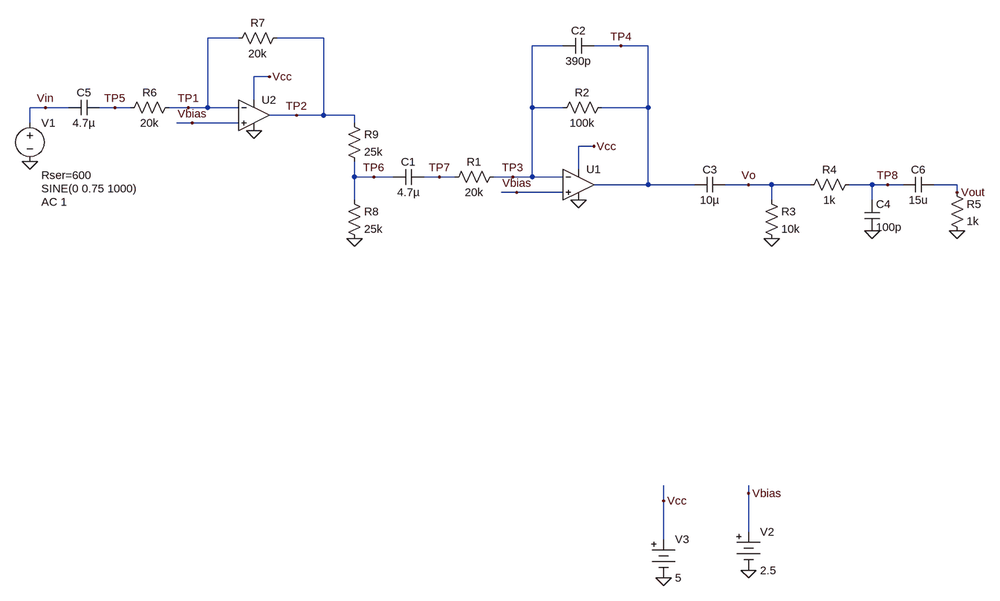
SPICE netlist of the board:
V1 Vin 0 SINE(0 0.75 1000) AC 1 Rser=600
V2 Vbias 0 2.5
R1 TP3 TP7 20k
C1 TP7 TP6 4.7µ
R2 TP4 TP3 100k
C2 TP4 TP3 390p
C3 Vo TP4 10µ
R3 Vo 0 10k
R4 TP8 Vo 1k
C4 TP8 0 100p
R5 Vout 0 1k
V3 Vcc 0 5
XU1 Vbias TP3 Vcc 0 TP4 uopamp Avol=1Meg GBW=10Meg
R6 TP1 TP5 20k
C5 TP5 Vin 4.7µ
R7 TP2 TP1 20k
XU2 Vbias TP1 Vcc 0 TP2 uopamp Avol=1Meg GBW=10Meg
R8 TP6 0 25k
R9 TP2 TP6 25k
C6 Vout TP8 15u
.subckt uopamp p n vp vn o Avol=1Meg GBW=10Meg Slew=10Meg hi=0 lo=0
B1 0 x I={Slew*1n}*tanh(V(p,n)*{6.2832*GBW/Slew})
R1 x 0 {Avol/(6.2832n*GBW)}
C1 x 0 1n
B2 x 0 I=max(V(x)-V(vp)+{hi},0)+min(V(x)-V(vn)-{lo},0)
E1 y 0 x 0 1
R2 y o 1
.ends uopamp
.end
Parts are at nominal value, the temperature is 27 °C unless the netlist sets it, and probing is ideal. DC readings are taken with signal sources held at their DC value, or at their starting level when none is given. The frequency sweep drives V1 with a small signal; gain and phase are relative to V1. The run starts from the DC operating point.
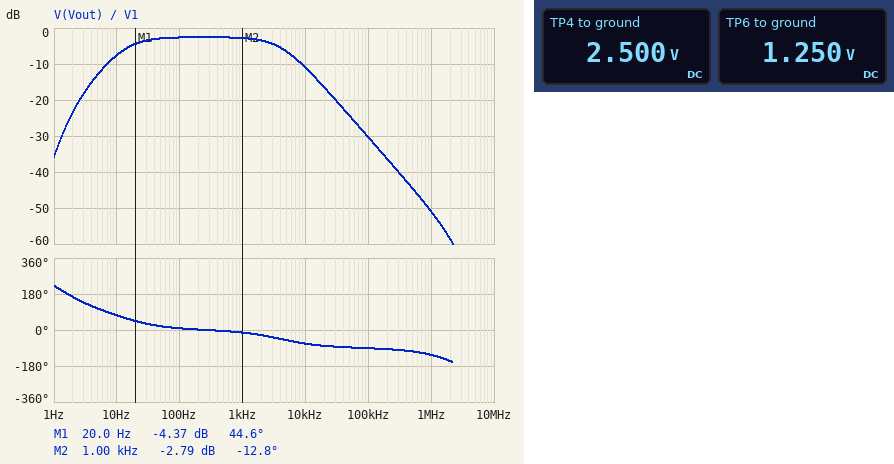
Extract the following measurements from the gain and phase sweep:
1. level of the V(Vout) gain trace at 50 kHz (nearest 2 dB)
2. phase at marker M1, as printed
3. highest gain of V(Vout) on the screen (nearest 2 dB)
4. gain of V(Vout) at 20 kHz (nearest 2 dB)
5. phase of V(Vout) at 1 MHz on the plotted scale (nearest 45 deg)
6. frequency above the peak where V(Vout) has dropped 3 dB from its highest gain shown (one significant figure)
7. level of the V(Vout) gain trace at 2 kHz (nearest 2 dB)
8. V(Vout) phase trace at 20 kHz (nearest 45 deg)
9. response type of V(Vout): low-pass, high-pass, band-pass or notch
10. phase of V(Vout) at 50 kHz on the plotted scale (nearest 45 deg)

-24 dB
44.6 deg
-2 dB
-16 dB
-135 deg
4 kHz
-4 dB
-90 deg
band-pass
-90 deg
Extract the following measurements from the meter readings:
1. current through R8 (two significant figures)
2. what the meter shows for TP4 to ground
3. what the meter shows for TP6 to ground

50 µA
2.500 V
1.250 V
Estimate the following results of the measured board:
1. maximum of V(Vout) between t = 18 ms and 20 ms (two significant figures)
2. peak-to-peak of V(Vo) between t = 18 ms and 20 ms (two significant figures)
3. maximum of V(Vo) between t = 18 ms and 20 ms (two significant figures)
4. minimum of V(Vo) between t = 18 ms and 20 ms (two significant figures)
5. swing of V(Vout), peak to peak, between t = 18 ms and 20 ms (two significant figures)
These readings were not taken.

540 mV
2.2 V
1.1 V
-1.1 V
1.1 V
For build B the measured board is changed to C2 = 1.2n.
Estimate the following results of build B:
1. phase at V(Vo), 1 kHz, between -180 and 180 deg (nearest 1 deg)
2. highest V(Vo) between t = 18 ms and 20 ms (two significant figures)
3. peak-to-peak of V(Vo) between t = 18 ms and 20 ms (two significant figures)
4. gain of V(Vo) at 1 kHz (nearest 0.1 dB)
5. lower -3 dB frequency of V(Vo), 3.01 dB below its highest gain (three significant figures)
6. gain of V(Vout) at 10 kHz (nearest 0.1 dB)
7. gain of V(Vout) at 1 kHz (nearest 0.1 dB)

-36 deg
890 mV
1.8 V
1.5 dB
12.2 Hz
-20.2 dB
-4.5 dB
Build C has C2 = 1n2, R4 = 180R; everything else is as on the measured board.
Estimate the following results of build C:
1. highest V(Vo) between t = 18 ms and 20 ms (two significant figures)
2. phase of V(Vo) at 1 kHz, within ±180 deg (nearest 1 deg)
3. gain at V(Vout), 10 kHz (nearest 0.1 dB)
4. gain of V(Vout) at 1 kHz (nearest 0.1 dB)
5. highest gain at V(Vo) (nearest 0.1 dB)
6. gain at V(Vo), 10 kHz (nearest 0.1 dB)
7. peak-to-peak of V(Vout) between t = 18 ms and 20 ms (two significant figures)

890 mV
-36 deg
-15.6 dB
0.1 dB
3.3 dB
-14.1 dB
1.5 V
